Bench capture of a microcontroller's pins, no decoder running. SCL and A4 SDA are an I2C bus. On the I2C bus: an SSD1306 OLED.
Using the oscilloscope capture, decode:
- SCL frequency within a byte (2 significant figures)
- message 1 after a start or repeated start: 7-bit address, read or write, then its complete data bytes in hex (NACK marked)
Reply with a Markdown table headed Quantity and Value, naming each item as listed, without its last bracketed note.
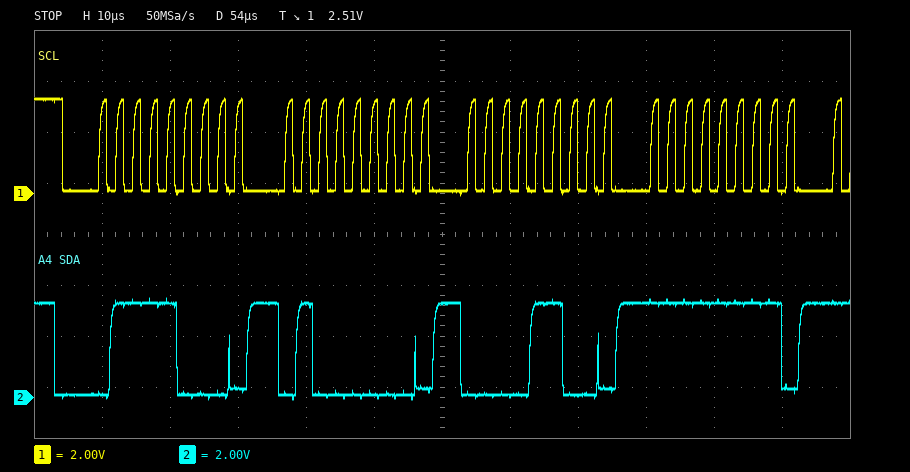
| Quantity | Value |
|---|---|
| SCL frequency within a byte | 400 kHz |
| message 1 after a start or repeated start: 7-bit address, read or write, then its complete data bytes in hex | 0x3C write: 40 0C FF |
